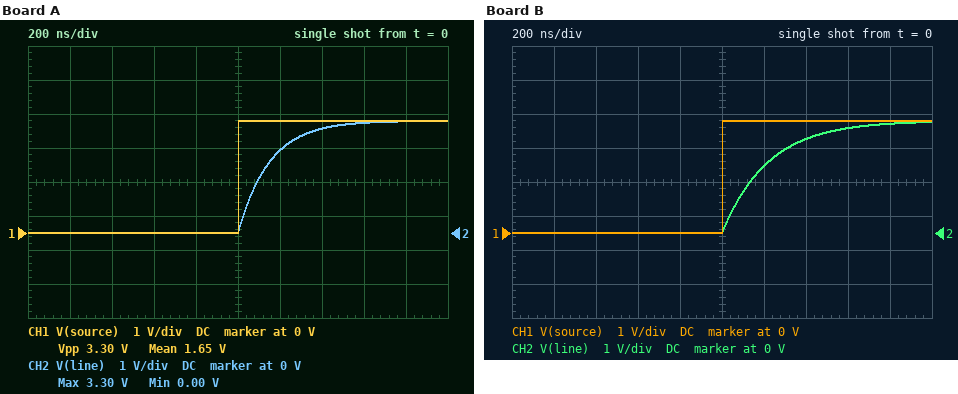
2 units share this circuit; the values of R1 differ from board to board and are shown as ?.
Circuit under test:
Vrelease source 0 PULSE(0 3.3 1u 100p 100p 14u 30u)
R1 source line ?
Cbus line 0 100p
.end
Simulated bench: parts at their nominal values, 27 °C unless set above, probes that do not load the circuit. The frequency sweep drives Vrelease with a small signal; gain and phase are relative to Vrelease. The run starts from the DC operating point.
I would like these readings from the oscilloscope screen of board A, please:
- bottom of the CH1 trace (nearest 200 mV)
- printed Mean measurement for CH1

0 V
1.65 V
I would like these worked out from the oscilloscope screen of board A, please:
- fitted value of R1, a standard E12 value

1.5 kΩ
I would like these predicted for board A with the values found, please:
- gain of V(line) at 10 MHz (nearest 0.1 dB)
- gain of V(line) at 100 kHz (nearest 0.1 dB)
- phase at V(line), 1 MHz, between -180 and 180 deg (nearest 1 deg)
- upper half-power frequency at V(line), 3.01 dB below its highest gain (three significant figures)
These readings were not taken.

-19.5 dB
0 dB
-43 deg
1.06 MHz
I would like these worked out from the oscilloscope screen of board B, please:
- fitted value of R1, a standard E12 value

2.2 kΩ
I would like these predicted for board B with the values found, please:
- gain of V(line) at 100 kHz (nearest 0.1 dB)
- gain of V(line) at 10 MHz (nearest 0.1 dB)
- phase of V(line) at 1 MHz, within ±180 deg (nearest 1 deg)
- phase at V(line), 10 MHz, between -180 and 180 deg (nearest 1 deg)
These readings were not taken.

-0.1 dB
-22.8 dB
-54 deg
-86 deg
